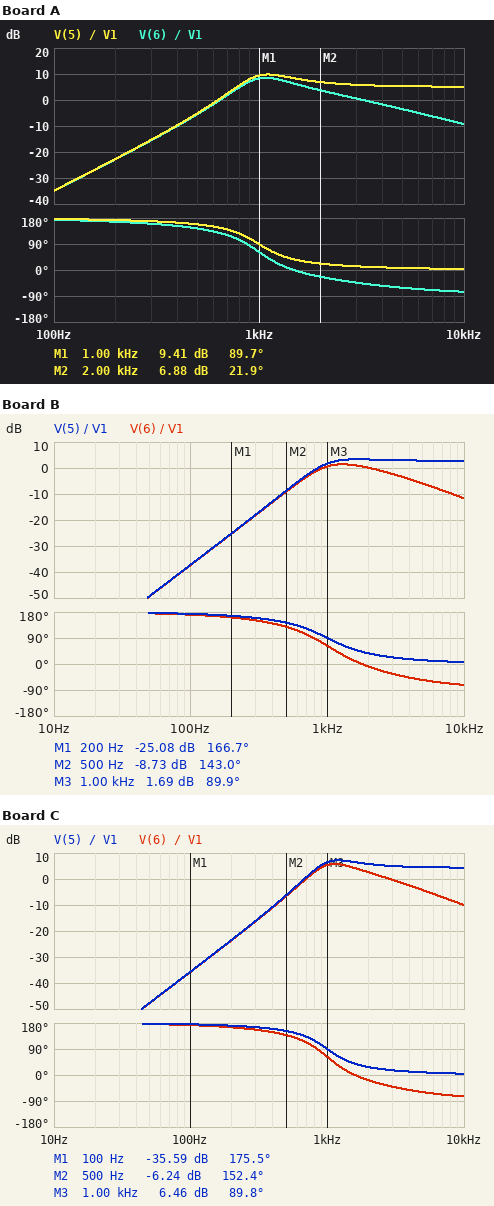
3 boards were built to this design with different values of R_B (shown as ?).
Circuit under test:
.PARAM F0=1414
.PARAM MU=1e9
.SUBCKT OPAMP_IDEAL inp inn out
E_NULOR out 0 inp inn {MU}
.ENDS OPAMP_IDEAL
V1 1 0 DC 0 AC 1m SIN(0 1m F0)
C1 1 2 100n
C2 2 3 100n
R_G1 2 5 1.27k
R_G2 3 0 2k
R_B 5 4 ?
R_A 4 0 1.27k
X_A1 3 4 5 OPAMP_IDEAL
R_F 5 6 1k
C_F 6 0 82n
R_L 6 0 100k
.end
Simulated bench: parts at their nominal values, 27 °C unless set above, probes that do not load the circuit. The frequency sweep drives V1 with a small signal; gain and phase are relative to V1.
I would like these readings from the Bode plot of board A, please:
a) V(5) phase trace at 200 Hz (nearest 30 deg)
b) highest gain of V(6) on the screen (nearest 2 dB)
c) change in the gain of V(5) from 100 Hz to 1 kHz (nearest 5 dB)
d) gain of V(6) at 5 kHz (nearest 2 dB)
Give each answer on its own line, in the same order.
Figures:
180 deg
8 dB
45 dB
-4 dB
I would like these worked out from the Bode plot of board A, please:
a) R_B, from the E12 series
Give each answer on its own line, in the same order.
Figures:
1 kΩ
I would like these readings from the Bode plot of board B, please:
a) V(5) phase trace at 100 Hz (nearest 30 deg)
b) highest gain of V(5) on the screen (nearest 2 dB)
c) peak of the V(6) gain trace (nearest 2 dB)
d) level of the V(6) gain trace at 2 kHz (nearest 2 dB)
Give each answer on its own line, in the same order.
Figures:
180 deg
4 dB
2 dB
0 dB
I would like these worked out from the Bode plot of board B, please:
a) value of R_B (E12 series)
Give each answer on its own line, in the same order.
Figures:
470 Ω
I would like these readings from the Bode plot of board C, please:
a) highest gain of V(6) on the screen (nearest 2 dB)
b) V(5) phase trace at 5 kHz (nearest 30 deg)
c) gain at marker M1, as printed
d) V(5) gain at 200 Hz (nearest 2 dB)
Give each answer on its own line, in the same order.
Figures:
6 dB
0 deg
-35.59 dB
-24 dB
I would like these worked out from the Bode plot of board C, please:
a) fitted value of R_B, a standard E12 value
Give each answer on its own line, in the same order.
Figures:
820 Ω
